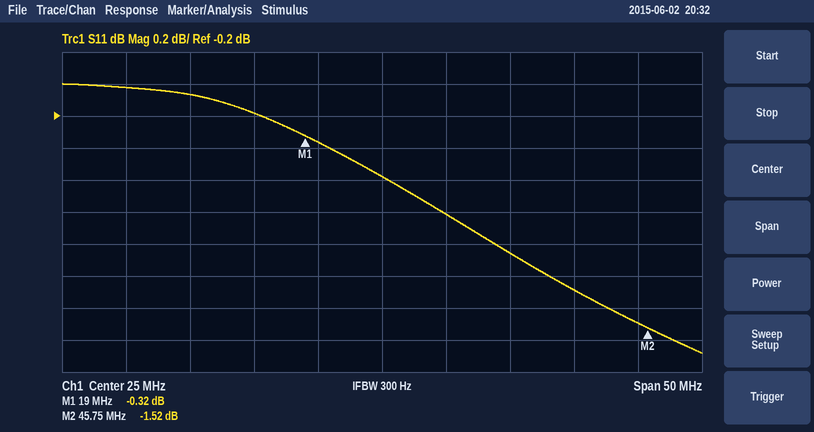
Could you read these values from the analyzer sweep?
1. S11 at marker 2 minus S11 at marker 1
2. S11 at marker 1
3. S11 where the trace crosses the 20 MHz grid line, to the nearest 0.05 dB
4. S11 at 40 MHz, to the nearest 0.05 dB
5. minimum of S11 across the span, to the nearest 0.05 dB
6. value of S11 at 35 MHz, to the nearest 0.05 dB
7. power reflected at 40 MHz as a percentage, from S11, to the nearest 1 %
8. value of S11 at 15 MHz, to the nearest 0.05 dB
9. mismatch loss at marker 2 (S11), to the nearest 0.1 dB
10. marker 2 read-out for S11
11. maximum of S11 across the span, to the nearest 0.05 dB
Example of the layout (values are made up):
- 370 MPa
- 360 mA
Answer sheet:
- -1.20 dB
- -0.32 dB
- -0.35 dB
- -1.30 dB
- -1.70 dB
- -1.05 dB
- 74 %
- -0.20 dB
- 5.3 dB
- -1.52 dB
- 0.00 dB
